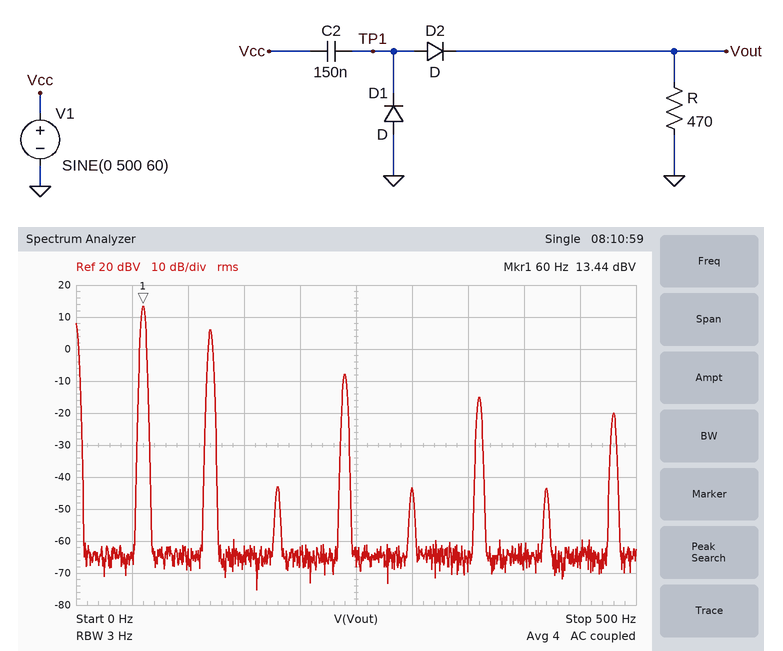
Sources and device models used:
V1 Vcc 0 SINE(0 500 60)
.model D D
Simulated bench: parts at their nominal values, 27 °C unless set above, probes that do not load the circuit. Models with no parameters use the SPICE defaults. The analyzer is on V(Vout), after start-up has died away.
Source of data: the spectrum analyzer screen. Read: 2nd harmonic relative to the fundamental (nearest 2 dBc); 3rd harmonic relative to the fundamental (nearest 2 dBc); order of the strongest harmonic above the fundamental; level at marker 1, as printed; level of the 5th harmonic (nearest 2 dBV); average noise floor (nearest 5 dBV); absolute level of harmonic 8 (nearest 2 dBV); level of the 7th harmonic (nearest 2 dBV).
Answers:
-8 dBc
-56 dBc
2
13.44 dBV
-44 dBV
-65 dBV
-20 dBV
-44 dBV
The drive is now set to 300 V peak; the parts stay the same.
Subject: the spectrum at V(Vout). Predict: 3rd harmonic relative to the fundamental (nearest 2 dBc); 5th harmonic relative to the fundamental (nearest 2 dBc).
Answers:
-52 dBc
-52 dBc
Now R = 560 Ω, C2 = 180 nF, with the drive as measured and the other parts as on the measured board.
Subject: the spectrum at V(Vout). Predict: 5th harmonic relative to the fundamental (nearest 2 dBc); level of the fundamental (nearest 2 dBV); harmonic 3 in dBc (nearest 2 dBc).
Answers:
-58 dBc
16 dBV
-58 dBc
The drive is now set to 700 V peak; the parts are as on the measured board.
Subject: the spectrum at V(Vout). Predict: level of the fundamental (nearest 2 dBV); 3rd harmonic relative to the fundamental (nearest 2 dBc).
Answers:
16 dBV
-60 dBc
